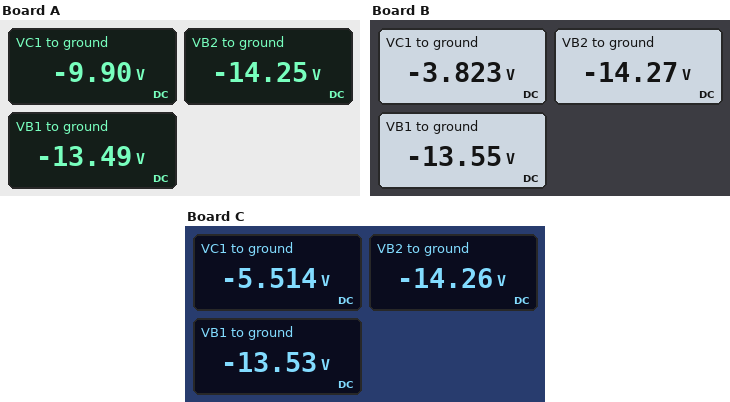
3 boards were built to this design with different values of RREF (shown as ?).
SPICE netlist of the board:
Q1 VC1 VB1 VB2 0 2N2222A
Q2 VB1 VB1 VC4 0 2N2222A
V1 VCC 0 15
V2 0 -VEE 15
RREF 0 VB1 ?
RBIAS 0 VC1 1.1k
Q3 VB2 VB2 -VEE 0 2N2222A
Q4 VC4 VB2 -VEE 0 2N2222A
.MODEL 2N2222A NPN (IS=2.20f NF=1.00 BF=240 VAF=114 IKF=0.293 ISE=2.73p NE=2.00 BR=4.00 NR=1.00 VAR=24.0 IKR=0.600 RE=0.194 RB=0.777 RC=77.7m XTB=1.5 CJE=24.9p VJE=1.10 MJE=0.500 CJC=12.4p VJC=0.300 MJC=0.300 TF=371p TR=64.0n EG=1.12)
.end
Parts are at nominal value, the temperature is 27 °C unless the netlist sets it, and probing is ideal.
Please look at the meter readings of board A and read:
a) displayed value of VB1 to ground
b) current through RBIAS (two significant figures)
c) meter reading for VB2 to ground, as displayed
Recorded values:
-13.49 V
9.0 mA
-14.25 V
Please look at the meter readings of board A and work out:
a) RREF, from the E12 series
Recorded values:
1.5 kΩ
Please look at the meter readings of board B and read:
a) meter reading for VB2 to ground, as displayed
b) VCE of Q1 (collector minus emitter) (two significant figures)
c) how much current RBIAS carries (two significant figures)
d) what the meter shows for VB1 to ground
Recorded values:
-14.27 V
10 V
3.5 mA
-13.55 V
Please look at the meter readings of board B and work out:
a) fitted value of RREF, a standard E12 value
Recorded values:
3.9 kΩ
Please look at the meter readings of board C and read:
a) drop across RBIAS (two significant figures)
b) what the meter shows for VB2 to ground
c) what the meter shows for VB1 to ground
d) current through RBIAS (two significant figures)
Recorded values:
5.5 V
-14.26 V
-13.53 V
5.0 mA
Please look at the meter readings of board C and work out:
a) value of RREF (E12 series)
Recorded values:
2.7 kΩ
